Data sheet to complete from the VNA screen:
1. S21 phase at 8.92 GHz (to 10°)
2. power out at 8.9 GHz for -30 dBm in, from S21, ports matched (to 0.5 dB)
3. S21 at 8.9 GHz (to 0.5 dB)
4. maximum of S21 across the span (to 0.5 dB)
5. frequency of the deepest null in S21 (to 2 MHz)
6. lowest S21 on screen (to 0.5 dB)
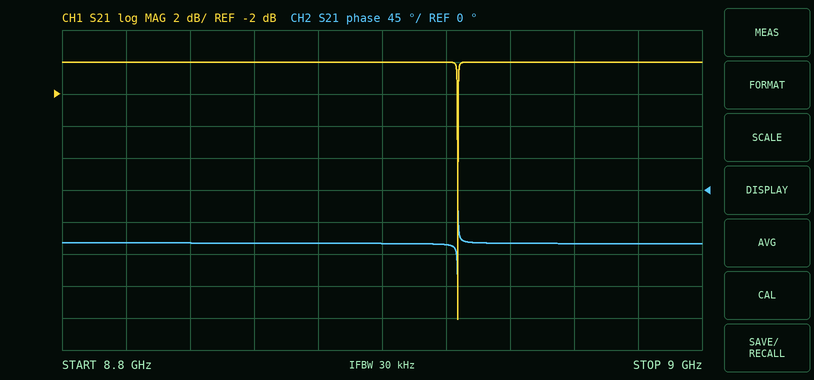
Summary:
-80°
-30.0 dBm
0.0 dB
0.0 dB
8.924 GHz
-16.0 dB
